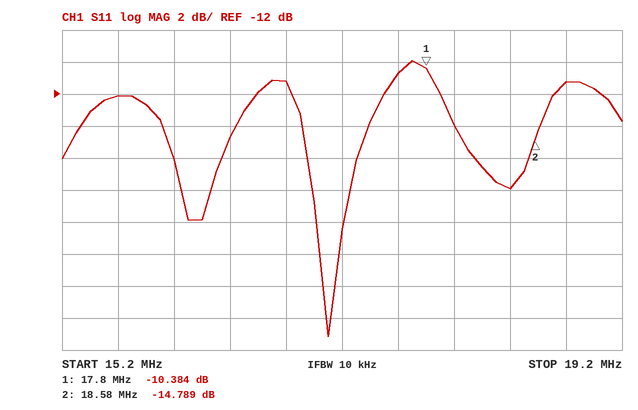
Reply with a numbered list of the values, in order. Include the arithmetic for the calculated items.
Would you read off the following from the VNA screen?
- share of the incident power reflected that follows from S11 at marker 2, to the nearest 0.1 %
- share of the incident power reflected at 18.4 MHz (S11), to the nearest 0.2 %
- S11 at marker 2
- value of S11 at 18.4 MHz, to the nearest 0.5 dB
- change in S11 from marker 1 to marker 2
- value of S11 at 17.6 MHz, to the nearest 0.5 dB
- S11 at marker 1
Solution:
1. 10^(-14.789/10) ≈ 3.3 %
2. 10^(-18/10) ≈ 1.6 %
3. -14.789 dB
4. -18.0 dB
5. -14.789 − (-10.384) = -4.405 dB
6. -10.5 dB
7. -10.384 dB
